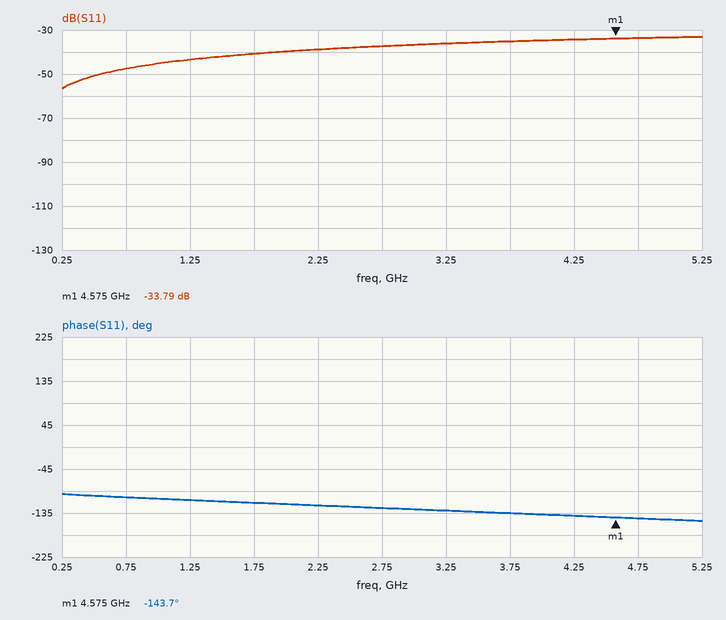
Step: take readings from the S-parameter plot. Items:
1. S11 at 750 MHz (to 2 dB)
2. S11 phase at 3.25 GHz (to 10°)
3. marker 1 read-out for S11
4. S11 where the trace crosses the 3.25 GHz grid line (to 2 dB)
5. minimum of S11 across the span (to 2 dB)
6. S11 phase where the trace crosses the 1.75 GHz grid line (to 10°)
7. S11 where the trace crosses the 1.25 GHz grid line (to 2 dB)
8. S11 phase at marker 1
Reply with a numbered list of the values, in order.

1. -48 dB
2. -130°
3. -33.79 dB
4. -36 dB
5. -56 dB
6. -110°
7. -44 dB
8. -143.7°
